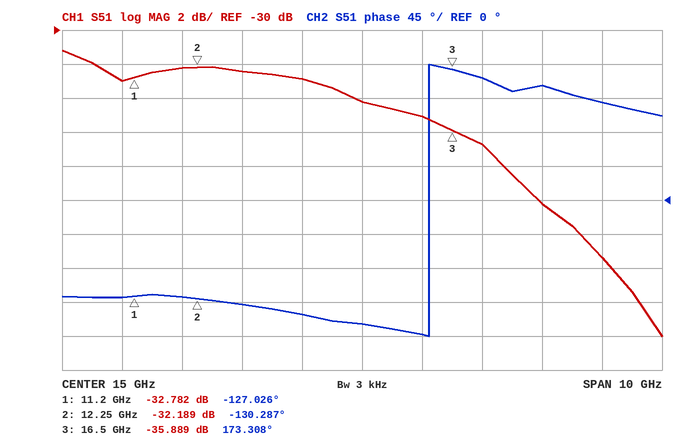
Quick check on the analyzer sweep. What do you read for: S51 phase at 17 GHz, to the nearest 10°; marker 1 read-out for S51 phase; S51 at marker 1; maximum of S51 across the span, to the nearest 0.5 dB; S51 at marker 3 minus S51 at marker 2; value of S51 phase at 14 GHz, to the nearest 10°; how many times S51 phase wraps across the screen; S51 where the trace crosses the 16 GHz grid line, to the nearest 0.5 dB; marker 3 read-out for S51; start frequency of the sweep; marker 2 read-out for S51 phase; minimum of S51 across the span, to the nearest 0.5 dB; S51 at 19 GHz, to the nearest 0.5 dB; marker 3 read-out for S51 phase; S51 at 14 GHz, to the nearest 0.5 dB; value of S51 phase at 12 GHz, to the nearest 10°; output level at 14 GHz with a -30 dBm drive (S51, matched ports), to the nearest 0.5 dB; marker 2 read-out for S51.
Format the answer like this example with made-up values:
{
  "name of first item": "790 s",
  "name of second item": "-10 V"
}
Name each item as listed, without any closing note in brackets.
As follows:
{
  "S51 phase at 17 GHz, to the nearest 10°": "160°",
  "marker 1 read-out for S51 phase": "-127.026°",
  "S51 at marker 1": "-32.782 dB",
  "maximum of S51 across the span, to the nearest 0.5 dB": "-31.0 dB",
  "S51 at marker 3 minus S51 at marker 2": "-3.700 dB",
  "value of S51 phase at 14 GHz, to the nearest 10°": "-150°",
  "how many times S51 phase wraps across the screen": "1",
  "S51 where the trace crosses the 16 GHz grid line, to the nearest 0.5 dB": "-35.0 dB",
  "marker 3 read-out for S51": "-35.889 dB",
  "start frequency of the sweep": "10 GHz",
  "marker 2 read-out for S51 phase": "-130.287°",
  "minimum of S51 across the span, to the nearest 0.5 dB": "-48.0 dB",
  "S51 at 19 GHz, to the nearest 0.5 dB": "-43.5 dB",
  "marker 3 read-out for S51 phase": "173.308°",
  "S51 at 14 GHz, to the nearest 0.5 dB": "-33.0 dB",
  "value of S51 phase at 12 GHz, to the nearest 10°": "-130°",
  "output level at 14 GHz with a -30 dBm drive (S51, matched ports), to the nearest 0.5 dB": "-63.0 dBm",
  "marker 2 read-out for S51": "-32.189 dB"
}
